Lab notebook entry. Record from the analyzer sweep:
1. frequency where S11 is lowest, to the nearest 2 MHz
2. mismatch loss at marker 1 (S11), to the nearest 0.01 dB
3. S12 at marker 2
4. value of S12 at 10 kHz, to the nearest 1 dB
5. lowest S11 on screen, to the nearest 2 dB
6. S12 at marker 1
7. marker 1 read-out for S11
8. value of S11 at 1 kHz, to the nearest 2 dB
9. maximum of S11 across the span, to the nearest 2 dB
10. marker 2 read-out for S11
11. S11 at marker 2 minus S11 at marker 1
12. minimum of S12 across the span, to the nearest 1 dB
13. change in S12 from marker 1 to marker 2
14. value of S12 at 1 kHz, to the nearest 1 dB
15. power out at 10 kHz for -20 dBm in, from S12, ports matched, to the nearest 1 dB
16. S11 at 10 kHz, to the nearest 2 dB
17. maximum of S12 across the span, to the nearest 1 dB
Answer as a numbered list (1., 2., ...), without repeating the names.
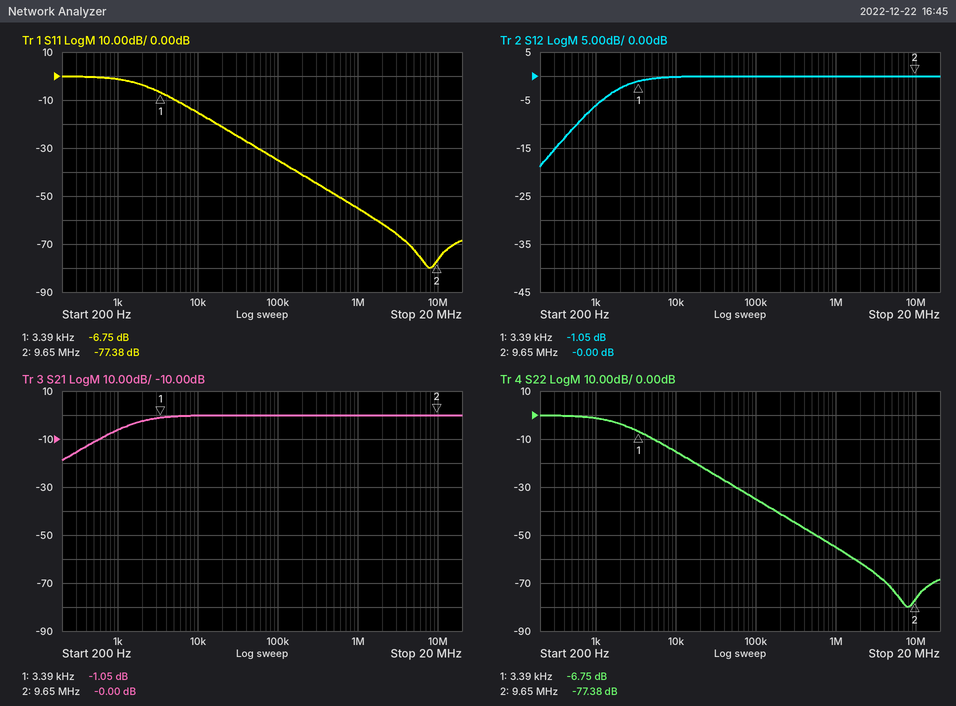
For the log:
1. 8 MHz
2. 1.03 dB
3. -0.00 dB
4. 0 dB
5. -80 dB
6. -1.05 dB
7. -6.75 dB
8. -2 dB
9. 0 dB
10. -77.38 dB
11. -70.63 dB
12. -19 dB
13. 1.05 dB
14. -6 dB
15. -20 dBm
16. -16 dB
17. 0 dB
